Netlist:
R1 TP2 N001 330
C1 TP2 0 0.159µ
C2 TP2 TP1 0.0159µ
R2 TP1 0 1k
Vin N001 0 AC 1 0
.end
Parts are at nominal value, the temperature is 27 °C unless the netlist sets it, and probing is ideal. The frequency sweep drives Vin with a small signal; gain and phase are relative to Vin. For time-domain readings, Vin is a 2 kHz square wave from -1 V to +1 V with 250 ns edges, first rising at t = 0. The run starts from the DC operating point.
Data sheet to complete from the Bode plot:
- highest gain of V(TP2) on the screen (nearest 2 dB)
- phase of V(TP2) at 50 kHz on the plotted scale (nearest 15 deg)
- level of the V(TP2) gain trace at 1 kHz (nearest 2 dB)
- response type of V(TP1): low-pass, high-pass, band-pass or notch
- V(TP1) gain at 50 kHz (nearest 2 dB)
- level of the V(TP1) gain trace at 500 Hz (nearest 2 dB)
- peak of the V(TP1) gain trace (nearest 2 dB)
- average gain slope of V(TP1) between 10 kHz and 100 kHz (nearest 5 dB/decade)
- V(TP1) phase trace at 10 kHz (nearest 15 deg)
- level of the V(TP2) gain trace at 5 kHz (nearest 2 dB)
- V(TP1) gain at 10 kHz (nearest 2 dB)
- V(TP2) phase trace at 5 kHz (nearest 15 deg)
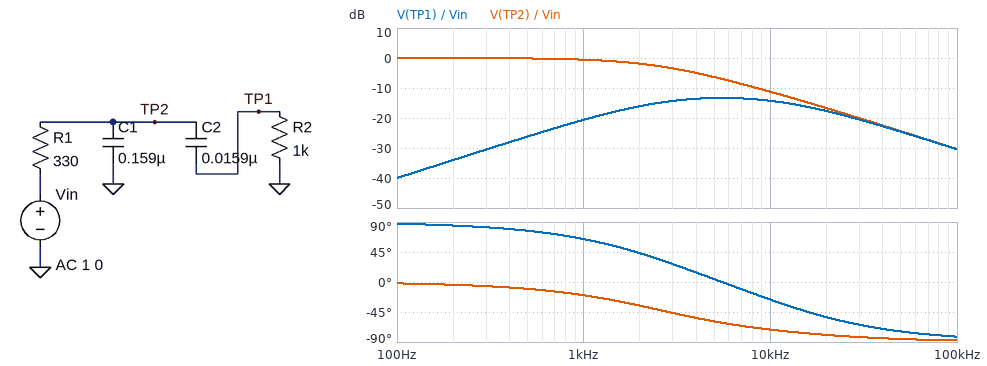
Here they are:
0 dB
-90 deg
0 dB
band-pass
-24 dB
-26 dB
-14 dB
-15 dB/decade
-30 deg
-6 dB
-14 dB
-60 deg
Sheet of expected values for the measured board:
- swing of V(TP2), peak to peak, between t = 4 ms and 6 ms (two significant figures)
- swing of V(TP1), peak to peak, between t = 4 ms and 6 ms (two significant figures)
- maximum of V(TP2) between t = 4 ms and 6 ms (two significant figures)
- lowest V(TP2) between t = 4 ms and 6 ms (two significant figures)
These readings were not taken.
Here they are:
1.9 V
670 mV
970 mV
-970 mV
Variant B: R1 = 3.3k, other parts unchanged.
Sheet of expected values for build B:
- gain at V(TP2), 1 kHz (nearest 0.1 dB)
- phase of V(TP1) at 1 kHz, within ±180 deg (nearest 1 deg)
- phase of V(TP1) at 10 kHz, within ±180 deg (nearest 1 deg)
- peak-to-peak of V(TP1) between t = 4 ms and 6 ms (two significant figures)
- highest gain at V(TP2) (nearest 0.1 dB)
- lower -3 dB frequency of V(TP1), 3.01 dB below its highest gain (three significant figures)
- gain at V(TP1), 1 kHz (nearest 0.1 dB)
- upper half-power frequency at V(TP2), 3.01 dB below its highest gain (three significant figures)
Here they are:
-11.5 dB
10 deg
-41 deg
60 mV
0 dB
262 Hz
-31.6 dB
275 Hz
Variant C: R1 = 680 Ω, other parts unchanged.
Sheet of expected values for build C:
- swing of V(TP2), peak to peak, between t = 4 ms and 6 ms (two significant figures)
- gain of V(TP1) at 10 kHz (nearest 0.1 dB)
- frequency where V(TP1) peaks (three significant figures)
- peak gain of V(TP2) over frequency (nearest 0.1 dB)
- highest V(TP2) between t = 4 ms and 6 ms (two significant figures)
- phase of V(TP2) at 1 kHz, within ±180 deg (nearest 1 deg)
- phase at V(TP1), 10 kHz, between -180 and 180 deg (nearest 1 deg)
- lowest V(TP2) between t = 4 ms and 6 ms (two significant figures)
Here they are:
1.6 V
-20.2 dB
3.84 kHz
0 dB
780 mV
-37 deg
-34 deg
-780 mV
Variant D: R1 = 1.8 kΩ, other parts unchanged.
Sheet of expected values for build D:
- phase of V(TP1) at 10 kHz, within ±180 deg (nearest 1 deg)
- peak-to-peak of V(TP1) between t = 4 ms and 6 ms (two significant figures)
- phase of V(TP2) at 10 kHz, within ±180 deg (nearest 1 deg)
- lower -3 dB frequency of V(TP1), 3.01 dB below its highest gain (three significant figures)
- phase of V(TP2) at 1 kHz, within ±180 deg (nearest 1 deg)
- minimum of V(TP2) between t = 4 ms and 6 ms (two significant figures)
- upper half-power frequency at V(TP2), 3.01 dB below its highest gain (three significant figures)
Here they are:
-39 deg
120 mV
-84 deg
463 Hz
-63 deg
-380 mV
503 Hz
